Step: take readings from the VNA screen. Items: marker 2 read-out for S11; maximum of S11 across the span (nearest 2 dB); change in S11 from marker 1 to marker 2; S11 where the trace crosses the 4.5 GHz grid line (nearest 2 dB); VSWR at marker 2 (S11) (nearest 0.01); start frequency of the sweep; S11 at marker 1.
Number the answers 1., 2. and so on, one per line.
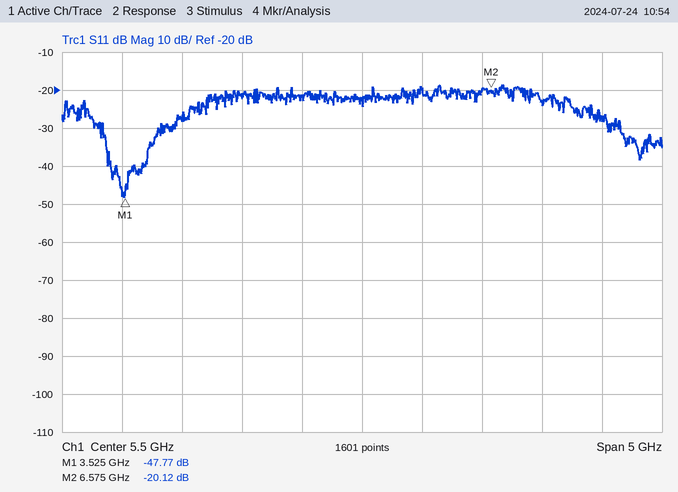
1. -20.12 dB
2. -18 dB
3. 27.65 dB
4. -22 dB
5. 1.22
6. 3 GHz
7. -47.77 dB
